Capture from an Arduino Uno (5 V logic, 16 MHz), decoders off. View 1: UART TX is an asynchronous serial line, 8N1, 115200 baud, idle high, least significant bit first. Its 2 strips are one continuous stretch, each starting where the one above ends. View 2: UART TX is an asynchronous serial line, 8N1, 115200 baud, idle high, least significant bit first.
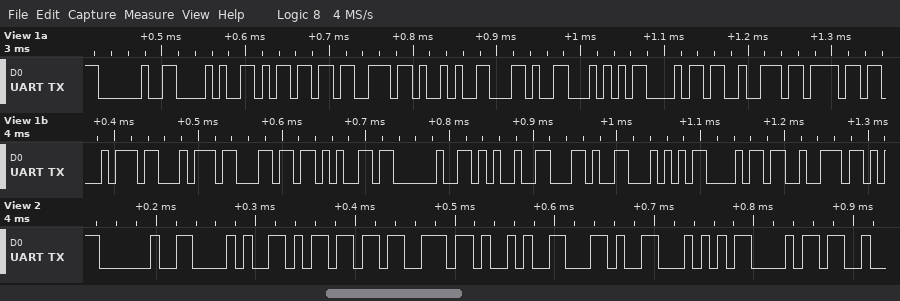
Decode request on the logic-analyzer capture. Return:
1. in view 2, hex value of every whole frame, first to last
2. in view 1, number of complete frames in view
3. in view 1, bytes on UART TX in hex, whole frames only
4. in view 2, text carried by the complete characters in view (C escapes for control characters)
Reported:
20 28 6D 73 29 2C 54 68
20
20 28 6D 73 29 2C 54 68 72 6F 74 74 6C 65 20 25 2C 54 68 72
" (ms),Th"
